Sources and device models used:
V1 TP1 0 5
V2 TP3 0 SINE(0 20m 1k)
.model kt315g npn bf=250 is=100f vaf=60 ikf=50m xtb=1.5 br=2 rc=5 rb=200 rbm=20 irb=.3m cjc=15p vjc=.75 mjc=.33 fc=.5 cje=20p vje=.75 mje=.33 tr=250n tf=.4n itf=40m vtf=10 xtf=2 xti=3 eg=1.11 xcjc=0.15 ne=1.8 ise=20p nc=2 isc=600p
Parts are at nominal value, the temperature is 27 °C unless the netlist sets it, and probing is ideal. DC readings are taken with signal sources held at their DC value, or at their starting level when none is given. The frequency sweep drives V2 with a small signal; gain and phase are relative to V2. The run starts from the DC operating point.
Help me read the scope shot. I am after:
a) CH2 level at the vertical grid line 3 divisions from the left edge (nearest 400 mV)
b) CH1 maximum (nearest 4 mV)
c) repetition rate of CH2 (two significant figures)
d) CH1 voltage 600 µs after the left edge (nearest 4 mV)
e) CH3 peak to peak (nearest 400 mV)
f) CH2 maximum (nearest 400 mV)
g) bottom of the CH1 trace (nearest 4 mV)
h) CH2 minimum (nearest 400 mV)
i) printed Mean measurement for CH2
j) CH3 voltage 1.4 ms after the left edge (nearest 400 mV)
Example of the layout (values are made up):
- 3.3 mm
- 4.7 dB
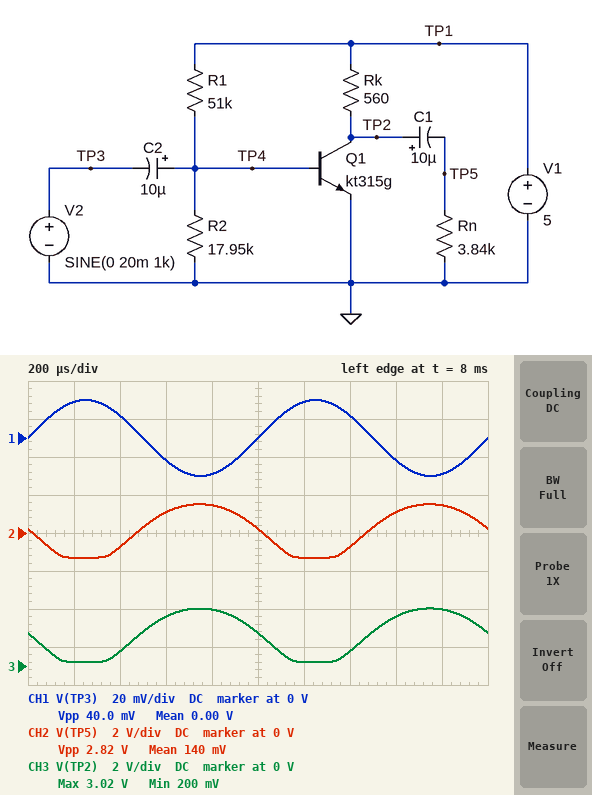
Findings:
- 1.2 V
- 20 mV
- 1.0 kHz
- -12 mV
- 2.8 V
- 1.6 V
- -20 mV
- -1.2 V
- 140 mV
- 800 mV
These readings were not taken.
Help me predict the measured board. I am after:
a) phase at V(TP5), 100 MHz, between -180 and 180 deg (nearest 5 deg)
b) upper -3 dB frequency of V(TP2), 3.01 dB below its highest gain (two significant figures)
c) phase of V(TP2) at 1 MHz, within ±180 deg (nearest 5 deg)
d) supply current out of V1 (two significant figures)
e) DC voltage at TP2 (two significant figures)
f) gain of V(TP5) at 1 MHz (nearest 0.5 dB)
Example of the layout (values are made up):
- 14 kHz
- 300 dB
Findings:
- 35 deg
- 3.7 MHz
- 165 deg
- 6.3 mA
- 1.5 V
- 38.0 dB
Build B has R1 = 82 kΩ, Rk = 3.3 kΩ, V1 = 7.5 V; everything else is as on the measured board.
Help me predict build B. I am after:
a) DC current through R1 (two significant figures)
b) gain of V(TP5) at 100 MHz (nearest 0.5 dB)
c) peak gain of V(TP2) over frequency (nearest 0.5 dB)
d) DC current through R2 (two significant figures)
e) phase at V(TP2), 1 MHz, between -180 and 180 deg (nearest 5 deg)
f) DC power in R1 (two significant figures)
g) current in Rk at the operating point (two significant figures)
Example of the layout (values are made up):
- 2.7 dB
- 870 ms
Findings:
- 84 µA
- -16.0 dB
- 15.0 dB
- 35 µA
- 115 deg
- 580 µW
- 2.2 mA
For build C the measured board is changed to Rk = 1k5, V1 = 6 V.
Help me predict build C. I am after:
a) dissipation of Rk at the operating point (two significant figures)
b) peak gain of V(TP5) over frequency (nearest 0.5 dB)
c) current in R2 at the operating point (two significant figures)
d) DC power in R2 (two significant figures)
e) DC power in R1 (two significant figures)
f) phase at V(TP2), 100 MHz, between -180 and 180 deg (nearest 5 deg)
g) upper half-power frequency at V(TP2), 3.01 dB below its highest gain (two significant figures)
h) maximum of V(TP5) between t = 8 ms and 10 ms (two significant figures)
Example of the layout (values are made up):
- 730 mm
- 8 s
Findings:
- 23 mW
- 13.5 dB
- 36 µA
- 23 µW
- 560 µW
- 45 deg
- 450 kHz
- 1.9 V
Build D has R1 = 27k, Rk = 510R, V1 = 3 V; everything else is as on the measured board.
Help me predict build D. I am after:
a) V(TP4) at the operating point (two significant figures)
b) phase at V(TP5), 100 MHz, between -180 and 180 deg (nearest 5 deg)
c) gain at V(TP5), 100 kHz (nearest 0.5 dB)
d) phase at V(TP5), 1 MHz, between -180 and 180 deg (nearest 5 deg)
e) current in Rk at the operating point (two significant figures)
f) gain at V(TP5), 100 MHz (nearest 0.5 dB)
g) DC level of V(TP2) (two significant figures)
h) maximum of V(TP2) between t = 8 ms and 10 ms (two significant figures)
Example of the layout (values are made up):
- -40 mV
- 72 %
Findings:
- 650 mV
- 55 deg
- 27.0 dB
- 130 deg
- 5.5 mA
- -10.0 dB
- 210 mV
- 1.7 V
